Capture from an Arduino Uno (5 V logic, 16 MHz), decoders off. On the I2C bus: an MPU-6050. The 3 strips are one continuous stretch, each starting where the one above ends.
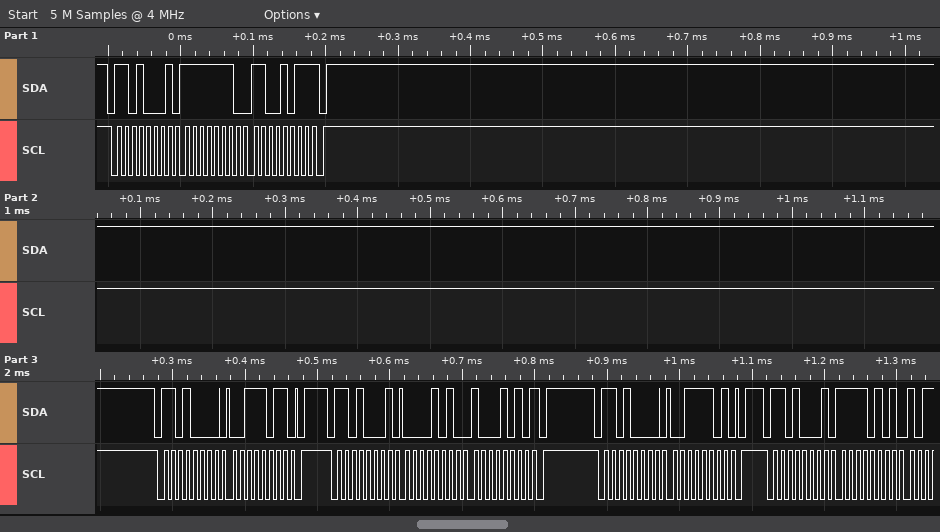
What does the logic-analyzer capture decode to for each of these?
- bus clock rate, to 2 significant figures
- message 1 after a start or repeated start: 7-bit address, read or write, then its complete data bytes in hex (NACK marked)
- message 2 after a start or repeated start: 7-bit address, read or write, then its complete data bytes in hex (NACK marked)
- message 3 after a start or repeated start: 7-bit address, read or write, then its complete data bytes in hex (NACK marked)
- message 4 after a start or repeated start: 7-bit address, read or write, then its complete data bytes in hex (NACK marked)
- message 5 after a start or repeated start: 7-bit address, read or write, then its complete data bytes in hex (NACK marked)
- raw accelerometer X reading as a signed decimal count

100 kHz
0x68 read: FE CB NACK
0x68 write: 3B
0x68 read: 0A 8A NACK
0x68 write: 3D
0x68 read: F5
2698
